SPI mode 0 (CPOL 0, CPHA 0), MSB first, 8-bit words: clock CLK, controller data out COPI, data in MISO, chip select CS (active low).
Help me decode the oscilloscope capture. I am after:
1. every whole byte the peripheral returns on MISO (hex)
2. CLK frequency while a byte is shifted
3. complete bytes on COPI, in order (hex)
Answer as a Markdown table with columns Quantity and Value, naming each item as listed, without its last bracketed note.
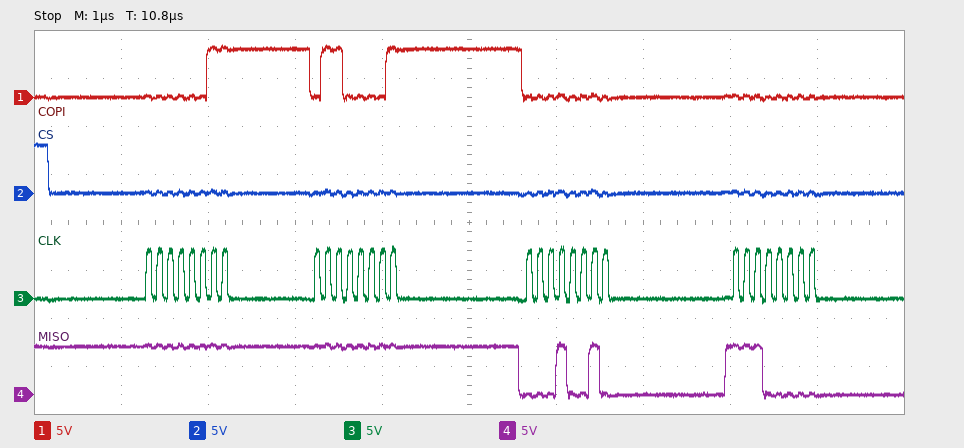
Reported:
| Quantity | Value |
|---|---|
| every whole byte the peripheral returns on MISO | 0xFF 0xFF 0x12 0xE0 |
| CLK frequency while a byte is shifted | 8 MHz |
| complete bytes on COPI, in order | 0x03 0x61 0x00 0x00 |
